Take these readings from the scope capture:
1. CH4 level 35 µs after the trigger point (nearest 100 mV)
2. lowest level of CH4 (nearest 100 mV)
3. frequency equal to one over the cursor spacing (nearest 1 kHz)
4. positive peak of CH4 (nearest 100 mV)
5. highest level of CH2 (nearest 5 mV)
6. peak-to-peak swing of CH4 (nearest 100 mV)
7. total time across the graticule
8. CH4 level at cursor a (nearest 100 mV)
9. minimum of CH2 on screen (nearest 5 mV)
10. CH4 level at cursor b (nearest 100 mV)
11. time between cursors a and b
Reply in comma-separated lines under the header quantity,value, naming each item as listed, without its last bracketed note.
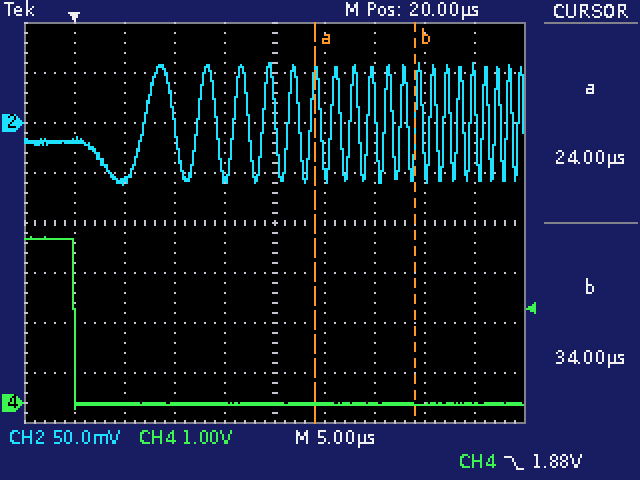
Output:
quantity,value
CH4 level 35 µs after the trigger point,0.0 V
lowest level of CH4,-100 mV
frequency equal to one over the cursor spacing,100 kHz
positive peak of CH4,3.3 V
highest level of CH2,60 mV
peak-to-peak swing of CH4,3.4 V
total time across the graticule,50 µs
CH4 level at cursor a,0.0 V
minimum of CH2 on screen,-60 mV
CH4 level at cursor b,0.0 V
time between cursors a and b,10.0 µs
